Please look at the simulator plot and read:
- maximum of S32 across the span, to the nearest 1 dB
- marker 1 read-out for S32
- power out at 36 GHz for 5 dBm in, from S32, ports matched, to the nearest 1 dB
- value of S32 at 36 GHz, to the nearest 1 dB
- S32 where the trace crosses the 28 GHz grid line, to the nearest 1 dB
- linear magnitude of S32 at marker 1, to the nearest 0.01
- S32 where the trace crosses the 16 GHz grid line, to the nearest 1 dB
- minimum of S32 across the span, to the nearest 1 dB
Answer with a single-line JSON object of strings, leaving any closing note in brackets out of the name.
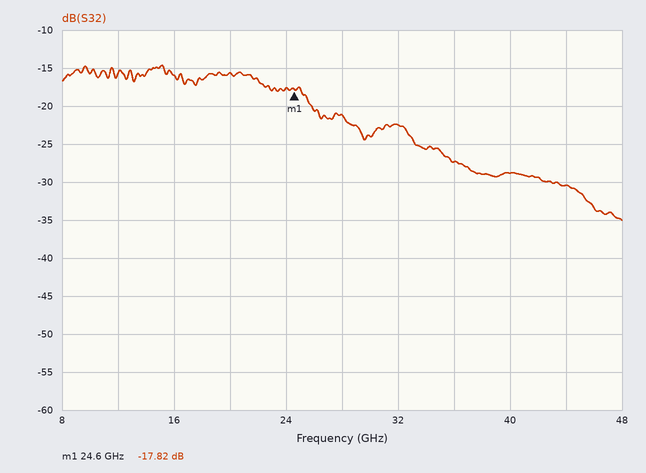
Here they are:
{"maximum of S32 across the span, to the nearest 1 dB": "-15 dB", "marker 1 read-out for S32": "-17.82 dB", "power out at 36 GHz for 5 dBm in, from S32, ports matched, to the nearest 1 dB": "-22 dBm", "value of S32 at 36 GHz, to the nearest 1 dB": "-27 dB", "S32 where the trace crosses the 28 GHz grid line, to the nearest 1 dB": "-21 dB", "linear magnitude of S32 at marker 1, to the nearest 0.01": "0.13", "S32 where the trace crosses the 16 GHz grid line, to the nearest 1 dB": "-16 dB", "minimum of S32 across the span, to the nearest 1 dB": "-35 dB"}
